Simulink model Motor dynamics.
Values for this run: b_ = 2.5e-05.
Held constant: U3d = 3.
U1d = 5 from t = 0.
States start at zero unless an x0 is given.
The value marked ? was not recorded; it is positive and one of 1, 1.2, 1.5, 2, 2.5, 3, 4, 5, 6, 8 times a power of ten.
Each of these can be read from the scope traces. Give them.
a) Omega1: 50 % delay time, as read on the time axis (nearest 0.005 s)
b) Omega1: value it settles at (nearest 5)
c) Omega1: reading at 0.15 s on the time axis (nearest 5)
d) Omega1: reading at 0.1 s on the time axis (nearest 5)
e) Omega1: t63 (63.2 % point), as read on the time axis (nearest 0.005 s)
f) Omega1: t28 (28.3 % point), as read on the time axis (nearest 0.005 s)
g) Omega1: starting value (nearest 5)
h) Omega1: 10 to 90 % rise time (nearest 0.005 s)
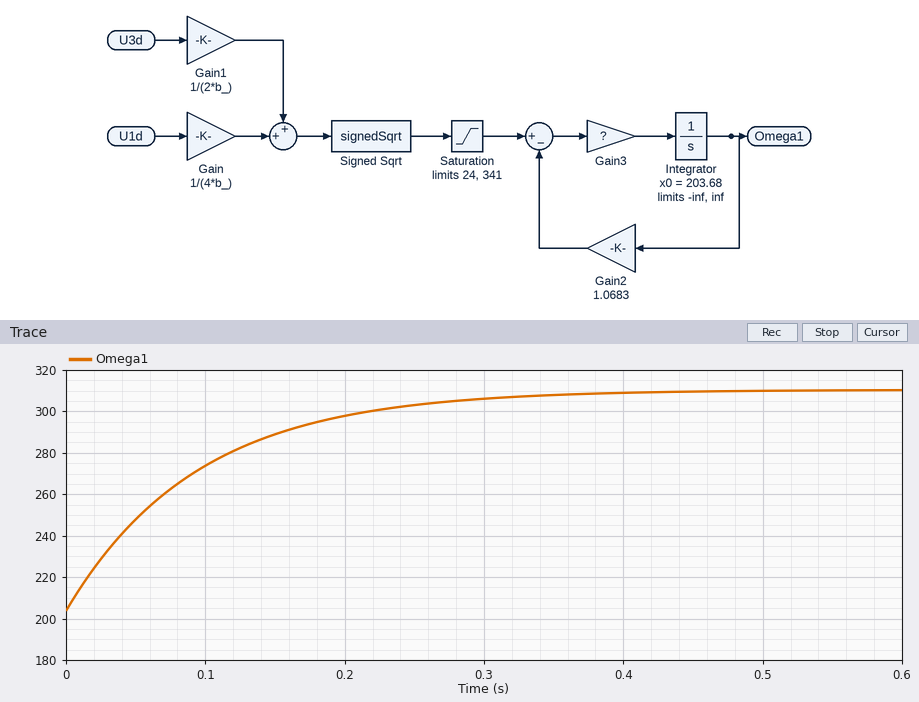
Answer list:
0.065 s
310
290
275
0.095 s
0.030 s
205
0.205 s
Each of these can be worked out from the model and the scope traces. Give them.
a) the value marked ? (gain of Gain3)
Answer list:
10
